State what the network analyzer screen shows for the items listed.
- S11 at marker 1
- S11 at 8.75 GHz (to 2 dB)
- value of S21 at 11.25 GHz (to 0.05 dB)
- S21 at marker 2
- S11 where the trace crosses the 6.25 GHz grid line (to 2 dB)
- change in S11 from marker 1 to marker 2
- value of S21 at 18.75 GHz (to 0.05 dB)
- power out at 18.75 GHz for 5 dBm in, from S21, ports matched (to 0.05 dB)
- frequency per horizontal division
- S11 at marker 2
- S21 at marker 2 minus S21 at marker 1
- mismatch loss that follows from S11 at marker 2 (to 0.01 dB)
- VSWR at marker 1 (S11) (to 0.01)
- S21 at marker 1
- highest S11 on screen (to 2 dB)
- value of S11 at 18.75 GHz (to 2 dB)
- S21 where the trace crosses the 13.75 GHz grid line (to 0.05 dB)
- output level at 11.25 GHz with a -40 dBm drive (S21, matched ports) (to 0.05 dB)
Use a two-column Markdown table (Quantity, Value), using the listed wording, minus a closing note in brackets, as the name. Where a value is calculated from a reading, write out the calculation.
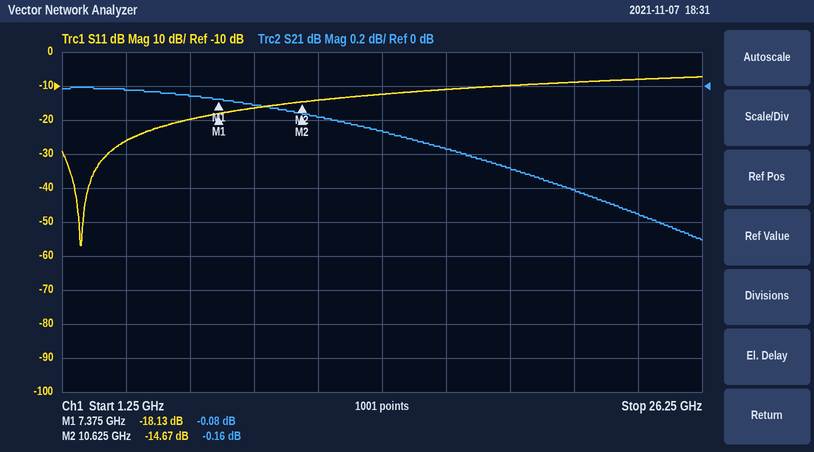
| Quantity | Value |
|---|---|
| S11 at marker 1 | -18.13 dB |
| S11 at 8.75 GHz | -16 dB |
| value of S21 at 11.25 GHz | -0.20 dB |
| S21 at marker 2 | -0.16 dB |
| S11 where the trace crosses the 6.25 GHz grid line | -20 dB |
| change in S11 from marker 1 to marker 2 | -14.67 − (-18.13) = 3.46 dB |
| value of S21 at 18.75 GHz | -0.50 dB |
| power out at 18.75 GHz for 5 dBm in, from S21, ports matched | 5 dBm + (-0.50 dB) = 4.50 dBm |
| frequency per horizontal division | 2.5 GHz |
| S11 at marker 2 | -14.67 dB |
| S21 at marker 2 minus S21 at marker 1 | -0.16 − (-0.08) = -0.08 dB |
| mismatch loss that follows from S11 at marker 2 | −10 log10(1 − 10^(-14.67/10)) ≈ 0.15 dB |
| VSWR at marker 1 (S11) | (1 + 0.1240)/(1 − 0.1240) ≈ 1.28 |
| S21 at marker 1 | -0.08 dB |
| highest S11 on screen | -8 dB |
| value of S11 at 18.75 GHz | -10 dB |
| S21 where the trace crosses the 13.75 GHz grid line | -0.25 dB |
| output level at 11.25 GHz with a -40 dBm drive (S21, matched ports) | -40 dBm + (-0.20 dB) = -40.20 dBm |
